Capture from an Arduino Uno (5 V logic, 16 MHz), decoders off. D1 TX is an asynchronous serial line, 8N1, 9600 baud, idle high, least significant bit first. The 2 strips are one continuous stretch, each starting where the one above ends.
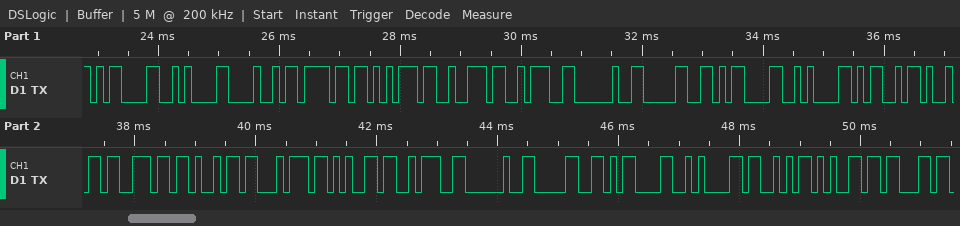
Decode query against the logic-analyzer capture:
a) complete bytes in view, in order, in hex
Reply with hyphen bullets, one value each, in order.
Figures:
- 0x0D 0x0A 0x48 0x6F 0x75 0x72 0x3A 0x20 0x30 0x0D 0x0A 0x4D 0x69 0x6E 0x69 0x74 0x65 0x3A 0x20 0x30 0x0D 0x0A 0x53 0x65 0x63
